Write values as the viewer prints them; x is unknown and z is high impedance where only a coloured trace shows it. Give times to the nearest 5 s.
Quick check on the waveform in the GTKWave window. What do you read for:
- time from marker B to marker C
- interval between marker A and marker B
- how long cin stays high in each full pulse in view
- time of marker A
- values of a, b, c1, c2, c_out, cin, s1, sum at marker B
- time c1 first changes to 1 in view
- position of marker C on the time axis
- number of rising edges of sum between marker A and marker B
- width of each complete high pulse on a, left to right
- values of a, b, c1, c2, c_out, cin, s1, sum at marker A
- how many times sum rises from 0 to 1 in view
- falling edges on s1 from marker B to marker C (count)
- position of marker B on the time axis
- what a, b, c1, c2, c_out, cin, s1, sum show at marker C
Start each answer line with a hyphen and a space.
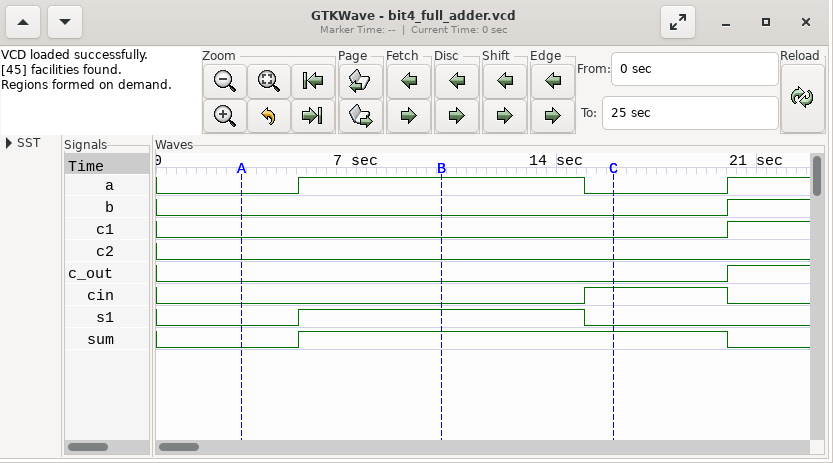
- 5 s
- 5 s
- 5 s
- 5 s
- a=1, b=0, c1=0, c2=0, c_out=0, cin=0, s1=1, sum=1
- 20 s
- 15 s
- 1
- 10 s
- a=0, b=0, c1=0, c2=0, c_out=0, cin=0, s1=0, sum=0
- 1
- 1
- 10 s
- a=0, b=0, c1=0, c2=0, c_out=0, cin=1, s1=0, sum=1
